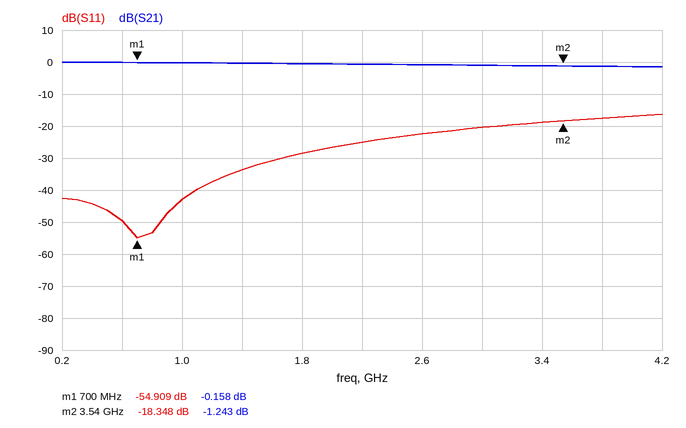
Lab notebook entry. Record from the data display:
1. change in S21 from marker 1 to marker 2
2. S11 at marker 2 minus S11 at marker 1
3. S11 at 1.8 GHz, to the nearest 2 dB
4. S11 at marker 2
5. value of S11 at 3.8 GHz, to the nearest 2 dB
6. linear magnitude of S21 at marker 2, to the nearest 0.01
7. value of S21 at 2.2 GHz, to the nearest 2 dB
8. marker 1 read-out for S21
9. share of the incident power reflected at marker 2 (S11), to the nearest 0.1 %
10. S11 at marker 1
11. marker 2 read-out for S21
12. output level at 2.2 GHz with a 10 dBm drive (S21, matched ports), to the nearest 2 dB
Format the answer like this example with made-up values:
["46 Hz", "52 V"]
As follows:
["-1.085 dB", "36.561 dB", "-28 dB", "-18.348 dB", "-18 dB", "0.87", "0 dB", "-0.158 dB", "1.5 %", "-54.909 dB", "-1.243 dB", "10 dBm"]
